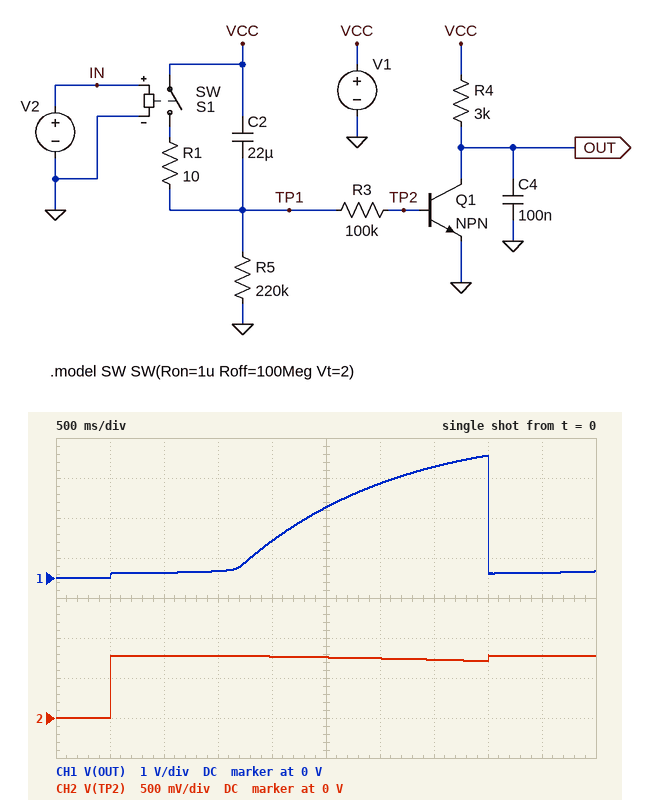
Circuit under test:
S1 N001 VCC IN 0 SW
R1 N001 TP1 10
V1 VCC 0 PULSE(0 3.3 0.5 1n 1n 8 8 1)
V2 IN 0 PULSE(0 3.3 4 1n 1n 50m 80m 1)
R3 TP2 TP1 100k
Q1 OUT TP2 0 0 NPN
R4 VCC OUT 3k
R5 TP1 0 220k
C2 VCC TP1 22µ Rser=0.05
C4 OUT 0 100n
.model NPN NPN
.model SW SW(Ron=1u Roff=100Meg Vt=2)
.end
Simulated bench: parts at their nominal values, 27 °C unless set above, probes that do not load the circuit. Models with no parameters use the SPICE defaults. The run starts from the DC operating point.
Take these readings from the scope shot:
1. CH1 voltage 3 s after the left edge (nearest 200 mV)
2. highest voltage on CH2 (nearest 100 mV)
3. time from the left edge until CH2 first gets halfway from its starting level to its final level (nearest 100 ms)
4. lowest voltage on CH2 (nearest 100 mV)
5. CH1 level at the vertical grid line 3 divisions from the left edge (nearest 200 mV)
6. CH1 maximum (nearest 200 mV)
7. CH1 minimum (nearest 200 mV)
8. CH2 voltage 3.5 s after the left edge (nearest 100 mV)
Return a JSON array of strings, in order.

["2.4 V", "800 mV", "500 ms", "0 V", "200 mV", "3.0 V", "0 V", "700 mV"]
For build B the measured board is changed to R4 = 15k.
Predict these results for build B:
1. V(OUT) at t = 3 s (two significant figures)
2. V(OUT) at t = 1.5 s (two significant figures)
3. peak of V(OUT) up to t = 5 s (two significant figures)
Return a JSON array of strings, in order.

["140 mV", "82 mV", "2.2 V"]
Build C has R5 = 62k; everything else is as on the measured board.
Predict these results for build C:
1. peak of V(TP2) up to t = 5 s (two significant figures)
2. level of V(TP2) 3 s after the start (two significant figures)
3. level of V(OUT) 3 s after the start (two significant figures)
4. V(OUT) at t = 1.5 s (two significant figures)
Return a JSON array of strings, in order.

["790 mV", "380 mV", "3.3 V", "1.9 V"]
